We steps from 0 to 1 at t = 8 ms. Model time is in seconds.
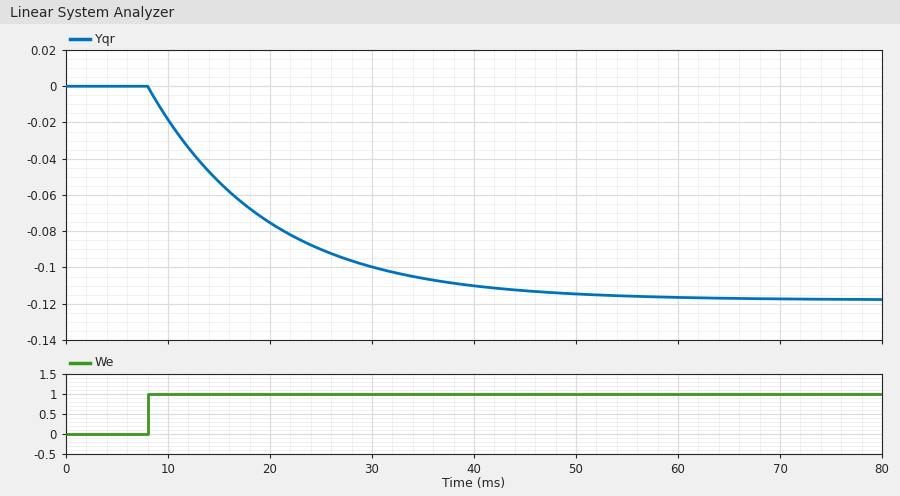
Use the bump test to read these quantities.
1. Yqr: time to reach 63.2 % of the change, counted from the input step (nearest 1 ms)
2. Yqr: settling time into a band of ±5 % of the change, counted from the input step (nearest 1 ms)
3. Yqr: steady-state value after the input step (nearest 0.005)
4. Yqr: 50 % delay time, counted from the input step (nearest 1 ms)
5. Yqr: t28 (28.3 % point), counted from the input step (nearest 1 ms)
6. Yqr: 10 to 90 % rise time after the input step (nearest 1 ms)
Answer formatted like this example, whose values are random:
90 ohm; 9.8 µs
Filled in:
12 ms; 35 ms; -0.120; 8 ms; 4 ms; 26 ms
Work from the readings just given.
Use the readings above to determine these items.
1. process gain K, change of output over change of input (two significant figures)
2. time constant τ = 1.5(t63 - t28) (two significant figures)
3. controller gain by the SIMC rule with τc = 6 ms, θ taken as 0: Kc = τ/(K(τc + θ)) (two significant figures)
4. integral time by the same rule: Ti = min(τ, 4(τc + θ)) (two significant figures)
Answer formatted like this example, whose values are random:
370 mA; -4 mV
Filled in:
-0.12; 12 ms; -17; 12 ms
